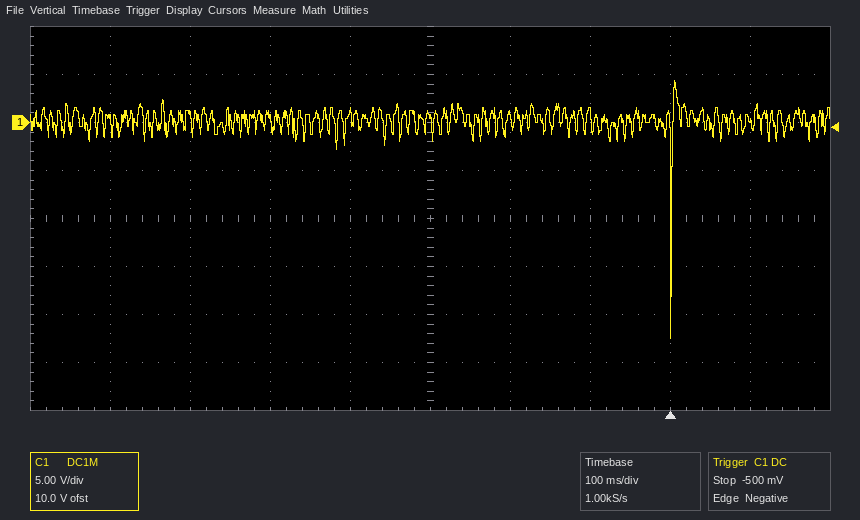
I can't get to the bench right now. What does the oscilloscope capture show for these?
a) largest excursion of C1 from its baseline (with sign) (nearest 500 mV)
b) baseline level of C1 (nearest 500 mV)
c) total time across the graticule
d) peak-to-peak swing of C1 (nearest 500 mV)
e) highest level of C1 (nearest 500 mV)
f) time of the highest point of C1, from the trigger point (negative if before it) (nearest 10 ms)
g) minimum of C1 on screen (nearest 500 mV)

-23.0 V
500 mV
1 s
27.0 V
4.5 V
+10 ms
-22.5 V
